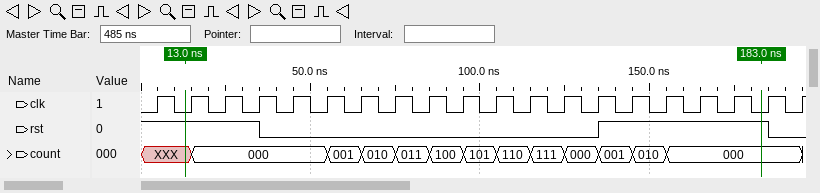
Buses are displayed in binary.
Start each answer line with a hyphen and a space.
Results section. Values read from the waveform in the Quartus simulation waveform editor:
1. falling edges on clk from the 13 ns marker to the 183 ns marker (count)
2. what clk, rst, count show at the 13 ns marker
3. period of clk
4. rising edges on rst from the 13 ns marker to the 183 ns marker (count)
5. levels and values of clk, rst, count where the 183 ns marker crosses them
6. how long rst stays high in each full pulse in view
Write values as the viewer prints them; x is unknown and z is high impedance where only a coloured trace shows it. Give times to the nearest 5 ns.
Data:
- 17
- clk=0, rst=1, count=XXX
- 10 ns
- 1
- clk=0, rst=1, count=000
- 50 ns
